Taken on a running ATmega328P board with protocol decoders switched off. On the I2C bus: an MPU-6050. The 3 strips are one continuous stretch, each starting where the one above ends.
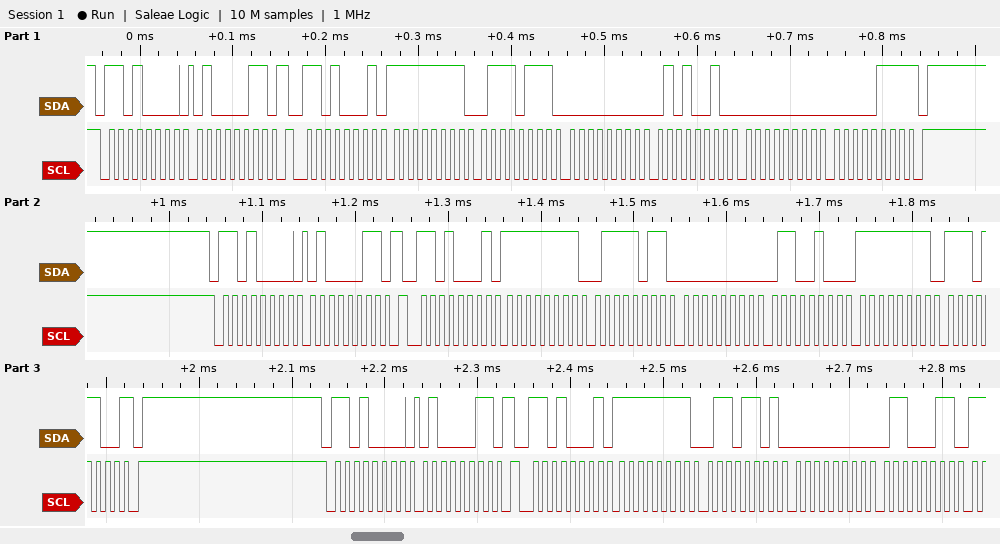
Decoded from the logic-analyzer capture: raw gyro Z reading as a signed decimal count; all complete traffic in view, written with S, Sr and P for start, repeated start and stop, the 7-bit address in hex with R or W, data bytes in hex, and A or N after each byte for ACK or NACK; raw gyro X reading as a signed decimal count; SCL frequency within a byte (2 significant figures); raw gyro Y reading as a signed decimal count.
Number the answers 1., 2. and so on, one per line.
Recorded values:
1. 7
2. S 68W A 43 A Sr 68R A FF A 77 A 00 A 52 A 00 A 07 N P S 68W A 43 A Sr 68R A FF A 7B A 00 A 64 A FF A EC N P S 68W A 43 A Sr 68R A FF A 6D A 00 A 63 A
3. -137
4. 100 kHz
5. 82
